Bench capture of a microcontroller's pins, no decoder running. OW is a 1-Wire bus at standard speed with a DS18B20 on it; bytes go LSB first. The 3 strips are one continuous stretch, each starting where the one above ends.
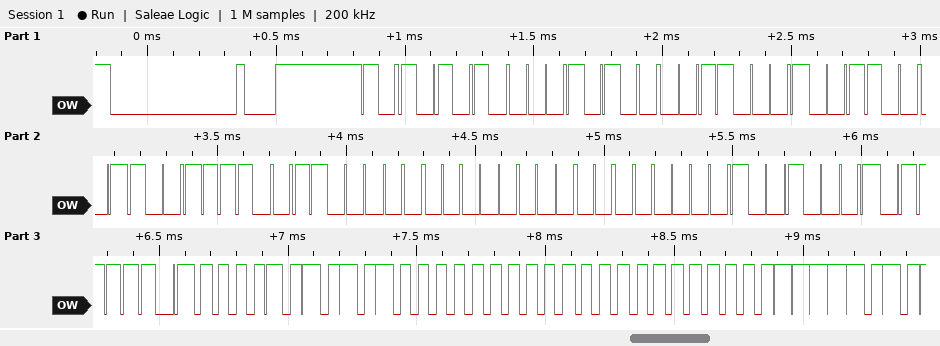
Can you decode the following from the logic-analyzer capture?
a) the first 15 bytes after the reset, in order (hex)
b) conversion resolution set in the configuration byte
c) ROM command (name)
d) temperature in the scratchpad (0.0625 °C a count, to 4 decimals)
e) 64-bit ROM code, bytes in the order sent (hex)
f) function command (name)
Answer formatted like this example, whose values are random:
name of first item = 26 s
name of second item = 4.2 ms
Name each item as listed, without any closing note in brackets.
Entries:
the first 15 bytes after the reset, in order = 55 28 8C 8C 79 06 00 00 89 BE 50 05 00 00 5F
conversion resolution set in the configuration byte = 11 bits
ROM command = Match ROM
temperature in the scratchpad = 85.0000 °C
64-bit ROM code, bytes in the order sent = 28 8C 8C 79 06 00 00 89
function command = Read Scratchpad
